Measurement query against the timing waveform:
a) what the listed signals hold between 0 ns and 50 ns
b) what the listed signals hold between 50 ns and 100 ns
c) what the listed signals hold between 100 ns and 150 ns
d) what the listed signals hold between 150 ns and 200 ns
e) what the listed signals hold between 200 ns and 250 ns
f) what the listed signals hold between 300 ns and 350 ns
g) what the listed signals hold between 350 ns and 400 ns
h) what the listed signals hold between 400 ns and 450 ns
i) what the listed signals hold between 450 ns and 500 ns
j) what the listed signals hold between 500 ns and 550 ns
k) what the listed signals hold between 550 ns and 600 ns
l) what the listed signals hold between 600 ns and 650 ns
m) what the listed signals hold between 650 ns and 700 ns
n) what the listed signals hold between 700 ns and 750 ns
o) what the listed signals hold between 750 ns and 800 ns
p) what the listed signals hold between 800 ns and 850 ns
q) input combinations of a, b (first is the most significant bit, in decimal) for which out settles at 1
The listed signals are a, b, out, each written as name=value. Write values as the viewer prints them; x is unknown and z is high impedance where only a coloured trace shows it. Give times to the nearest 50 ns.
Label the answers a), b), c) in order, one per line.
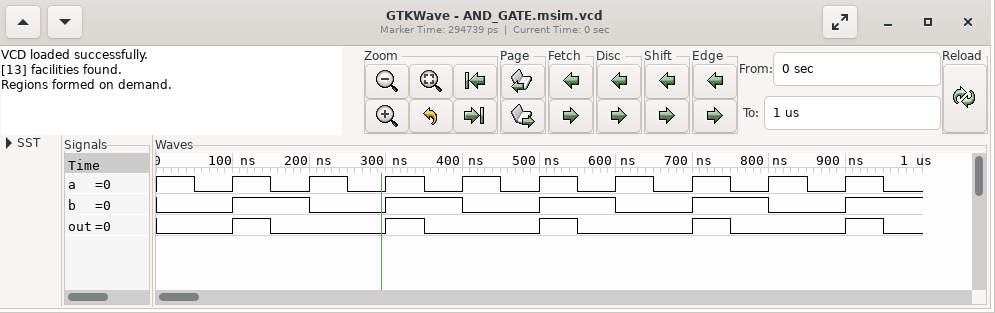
a) a=1, b=0, out=0
b) a=0, b=0, out=0
c) a=1, b=1, out=1
d) a=0, b=1, out=0
e) a=1, b=0, out=0
f) a=1, b=1, out=1
g) a=0, b=1, out=0
h) a=1, b=0, out=0
i) a=0, b=0, out=0
j) a=1, b=1, out=1
k) a=0, b=1, out=0
l) a=1, b=0, out=0
m) a=0, b=0, out=0
n) a=1, b=1, out=1
o) a=0, b=1, out=0
p) a=1, b=0, out=0
q) 3
